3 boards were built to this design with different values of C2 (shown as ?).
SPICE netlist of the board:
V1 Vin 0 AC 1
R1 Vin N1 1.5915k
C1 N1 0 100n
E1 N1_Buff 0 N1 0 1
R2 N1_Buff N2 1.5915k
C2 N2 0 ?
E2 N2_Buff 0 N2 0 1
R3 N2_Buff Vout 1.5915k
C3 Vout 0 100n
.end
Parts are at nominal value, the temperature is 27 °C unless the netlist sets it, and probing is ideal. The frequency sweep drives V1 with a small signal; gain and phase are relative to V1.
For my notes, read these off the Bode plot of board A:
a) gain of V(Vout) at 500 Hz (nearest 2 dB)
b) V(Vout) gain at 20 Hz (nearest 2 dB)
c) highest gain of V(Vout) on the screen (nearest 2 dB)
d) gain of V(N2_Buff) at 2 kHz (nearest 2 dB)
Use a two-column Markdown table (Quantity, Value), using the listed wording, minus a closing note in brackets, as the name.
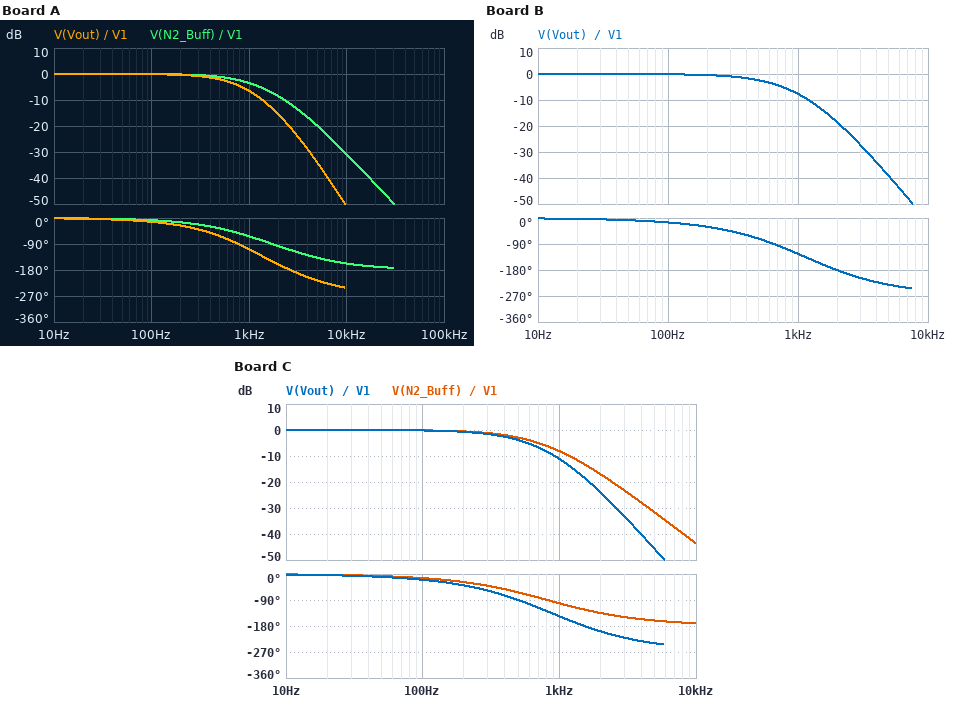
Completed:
| Quantity | Value |
|---|---|
| gain of V(Vout) at 500 Hz | -2 dB |
| V(Vout) gain at 20 Hz | 0 dB |
| highest gain of V(Vout) on the screen | 0 dB |
| gain of V(N2_Buff) at 2 kHz | -8 dB |
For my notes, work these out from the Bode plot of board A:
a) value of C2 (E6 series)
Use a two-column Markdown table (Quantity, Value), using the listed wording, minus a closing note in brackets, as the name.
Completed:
| Quantity | Value |
|---|---|
| value of C2 | 33 nF |
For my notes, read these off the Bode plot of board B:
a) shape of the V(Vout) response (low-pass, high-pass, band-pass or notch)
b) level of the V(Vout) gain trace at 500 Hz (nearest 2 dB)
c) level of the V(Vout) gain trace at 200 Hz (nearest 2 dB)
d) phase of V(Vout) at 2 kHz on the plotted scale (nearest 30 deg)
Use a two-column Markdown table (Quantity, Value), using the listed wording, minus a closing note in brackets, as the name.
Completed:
| Quantity | Value |
|---|---|
| shape of the V(Vout) response | low-pass |
| level of the V(Vout) gain trace at 500 Hz | -2 dB |
| level of the V(Vout) gain trace at 200 Hz | 0 dB |
| phase of V(Vout) at 2 kHz on the plotted scale | -180 deg |
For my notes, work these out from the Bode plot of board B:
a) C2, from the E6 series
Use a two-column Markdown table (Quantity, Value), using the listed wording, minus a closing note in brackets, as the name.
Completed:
| Quantity | Value |
|---|---|
| C2, from the E6 series | 68 nF |
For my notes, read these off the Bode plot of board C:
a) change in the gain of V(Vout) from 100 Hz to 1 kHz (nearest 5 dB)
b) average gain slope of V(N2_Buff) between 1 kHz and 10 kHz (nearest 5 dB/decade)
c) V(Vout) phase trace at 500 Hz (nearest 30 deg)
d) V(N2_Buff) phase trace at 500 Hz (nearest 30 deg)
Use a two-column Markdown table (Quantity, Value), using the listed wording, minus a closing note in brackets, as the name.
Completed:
| Quantity | Value |
|---|---|
| change in the gain of V(Vout) from 100 Hz to 1 kHz | -10 dB |
| average gain slope of V(N2_Buff) between 1 kHz and 10 kHz | -35 dB/decade |
| V(Vout) phase trace at 500 Hz | -90 deg |
| V(N2_Buff) phase trace at 500 Hz | -60 deg |
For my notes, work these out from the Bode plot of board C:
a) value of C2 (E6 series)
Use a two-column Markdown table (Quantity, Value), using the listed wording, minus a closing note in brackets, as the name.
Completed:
| Quantity | Value |
|---|---|
| value of C2 | 150 nF |
